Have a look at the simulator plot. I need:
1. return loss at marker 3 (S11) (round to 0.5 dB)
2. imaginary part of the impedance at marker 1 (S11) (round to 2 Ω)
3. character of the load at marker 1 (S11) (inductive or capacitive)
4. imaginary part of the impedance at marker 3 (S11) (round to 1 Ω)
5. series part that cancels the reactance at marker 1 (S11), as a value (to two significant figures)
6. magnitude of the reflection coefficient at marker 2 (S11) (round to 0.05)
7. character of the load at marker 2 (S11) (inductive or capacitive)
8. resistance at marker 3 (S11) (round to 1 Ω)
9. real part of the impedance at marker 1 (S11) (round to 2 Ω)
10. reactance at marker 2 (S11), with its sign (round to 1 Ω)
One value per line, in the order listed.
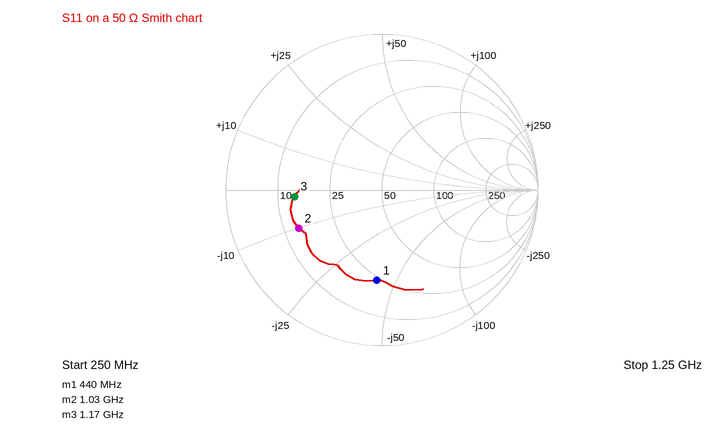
5.0 dB
-42 Ω
capacitive
-2 Ω
15 nH
0.60
capacitive
14 Ω
24 Ω
-10 Ω
